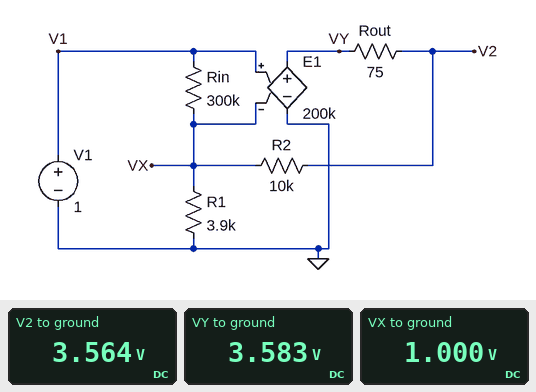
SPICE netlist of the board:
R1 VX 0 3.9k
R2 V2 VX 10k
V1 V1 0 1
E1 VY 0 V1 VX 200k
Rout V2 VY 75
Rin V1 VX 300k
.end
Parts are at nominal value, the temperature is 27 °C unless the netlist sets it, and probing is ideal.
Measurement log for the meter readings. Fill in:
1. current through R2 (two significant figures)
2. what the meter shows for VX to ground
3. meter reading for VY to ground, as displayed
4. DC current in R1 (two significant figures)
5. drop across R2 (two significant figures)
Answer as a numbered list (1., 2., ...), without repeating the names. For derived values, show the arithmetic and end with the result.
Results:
1. (3.564 V - 1 V) / 10 kΩ = 260 µA
2. 1.000 V
3. 3.583 V
4. (1 V) / 3.9 kΩ = 260 µA
5. 3.564 V - 1 V = 2.6 V
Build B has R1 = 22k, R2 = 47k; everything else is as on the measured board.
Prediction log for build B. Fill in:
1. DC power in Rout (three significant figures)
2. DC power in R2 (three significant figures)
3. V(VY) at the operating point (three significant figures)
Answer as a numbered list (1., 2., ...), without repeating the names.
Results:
1. 155 nW
2. 97.1 µW
3. 3.14 V
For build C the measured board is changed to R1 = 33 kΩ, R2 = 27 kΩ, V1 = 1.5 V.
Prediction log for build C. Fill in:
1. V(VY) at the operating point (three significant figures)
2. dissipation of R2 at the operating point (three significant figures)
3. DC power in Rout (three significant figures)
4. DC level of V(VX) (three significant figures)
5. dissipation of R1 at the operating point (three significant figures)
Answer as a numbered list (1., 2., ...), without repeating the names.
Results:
1. 2.73 V
2. 55.8 µW
3. 155 nW
4. 1.50 V
5. 68.2 µW
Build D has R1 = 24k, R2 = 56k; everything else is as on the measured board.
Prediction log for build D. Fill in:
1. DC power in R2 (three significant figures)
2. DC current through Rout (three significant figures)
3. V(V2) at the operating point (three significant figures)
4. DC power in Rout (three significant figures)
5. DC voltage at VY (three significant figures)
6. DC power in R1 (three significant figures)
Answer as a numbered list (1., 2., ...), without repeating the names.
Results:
1. 97.2 µW
2. 41.7 µA
3. 3.33 V
4. 130 nW
5. 3.34 V
6. 41.7 µW
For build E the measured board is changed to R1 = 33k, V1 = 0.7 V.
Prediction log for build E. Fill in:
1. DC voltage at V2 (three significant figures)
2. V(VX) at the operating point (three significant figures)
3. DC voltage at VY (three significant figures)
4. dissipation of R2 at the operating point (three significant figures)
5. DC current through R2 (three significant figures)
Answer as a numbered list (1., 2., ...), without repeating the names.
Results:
1. 912 mV
2. 700 mV
3. 914 mV
4. 4.50 µW
5. 21.2 µA
